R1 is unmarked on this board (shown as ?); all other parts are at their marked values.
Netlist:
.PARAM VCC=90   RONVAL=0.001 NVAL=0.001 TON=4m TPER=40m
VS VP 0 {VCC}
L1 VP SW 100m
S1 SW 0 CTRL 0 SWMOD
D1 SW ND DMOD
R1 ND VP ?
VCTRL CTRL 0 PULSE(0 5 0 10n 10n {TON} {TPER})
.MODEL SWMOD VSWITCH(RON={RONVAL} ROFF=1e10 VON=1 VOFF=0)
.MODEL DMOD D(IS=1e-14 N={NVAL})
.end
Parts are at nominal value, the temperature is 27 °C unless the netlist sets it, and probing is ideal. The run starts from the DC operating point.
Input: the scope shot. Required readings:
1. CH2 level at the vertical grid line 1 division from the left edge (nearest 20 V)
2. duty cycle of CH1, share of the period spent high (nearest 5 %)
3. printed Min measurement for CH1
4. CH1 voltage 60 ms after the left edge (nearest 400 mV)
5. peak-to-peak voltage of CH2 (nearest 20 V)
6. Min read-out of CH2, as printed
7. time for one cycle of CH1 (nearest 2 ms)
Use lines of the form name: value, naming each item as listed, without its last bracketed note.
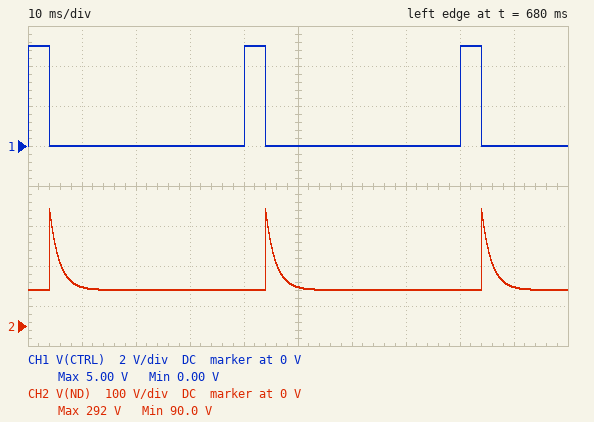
CH2 level at the vertical grid line 1 division from the left edge: 100 V
duty cycle of CH1, share of the period spent high: 10 %
printed Min measurement for CH1: 0.00 V
CH1 voltage 60 ms after the left edge: 0 V
peak-to-peak voltage of CH2: 200 V
Min read-out of CH2, as printed: 90.0 V
time for one cycle of CH1: 40 ms
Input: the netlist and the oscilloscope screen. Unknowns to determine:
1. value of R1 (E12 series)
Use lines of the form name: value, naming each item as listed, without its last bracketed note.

value of R1: 56 Ω
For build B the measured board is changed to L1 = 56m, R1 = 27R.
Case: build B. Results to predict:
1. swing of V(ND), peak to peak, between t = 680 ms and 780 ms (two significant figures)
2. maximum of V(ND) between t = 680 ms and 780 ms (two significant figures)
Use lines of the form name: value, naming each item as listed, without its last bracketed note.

swing of V(ND), peak to peak, between t = 680 ms and 780 ms: 170 V
maximum of V(ND) between t = 680 ms and 780 ms: 260 V
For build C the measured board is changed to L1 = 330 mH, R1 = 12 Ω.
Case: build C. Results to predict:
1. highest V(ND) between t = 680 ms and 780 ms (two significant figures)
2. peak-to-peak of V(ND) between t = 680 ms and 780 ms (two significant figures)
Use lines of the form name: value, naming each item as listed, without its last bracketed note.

highest V(ND) between t = 680 ms and 780 ms: 110 V
peak-to-peak of V(ND) between t = 680 ms and 780 ms: 18 V
